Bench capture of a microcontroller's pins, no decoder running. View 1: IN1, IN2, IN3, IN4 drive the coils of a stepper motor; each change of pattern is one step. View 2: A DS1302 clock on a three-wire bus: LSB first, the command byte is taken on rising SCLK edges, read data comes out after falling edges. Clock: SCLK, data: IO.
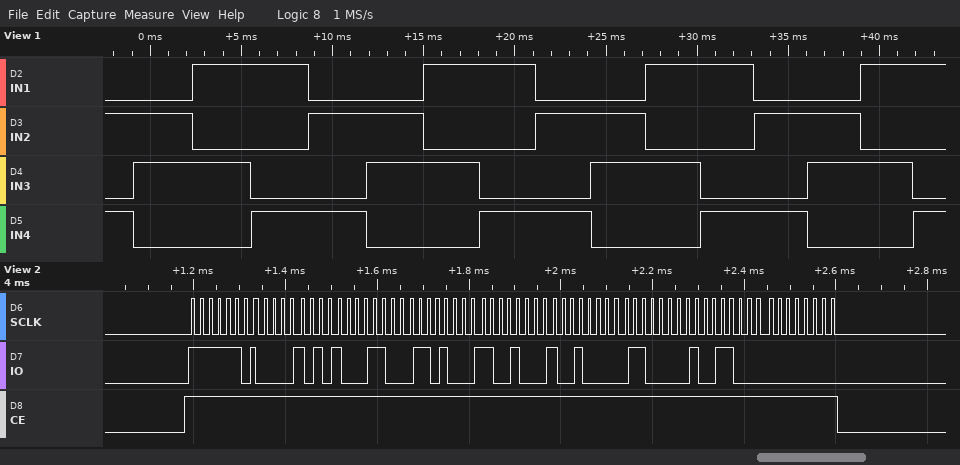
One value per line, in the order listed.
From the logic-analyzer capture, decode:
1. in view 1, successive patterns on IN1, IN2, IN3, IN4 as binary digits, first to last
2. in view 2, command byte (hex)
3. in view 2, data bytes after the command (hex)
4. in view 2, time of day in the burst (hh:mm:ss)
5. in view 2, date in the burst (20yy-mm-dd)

0101 0110 1010 1001 0101 0110 1010 1001 0101 0110 1010 1001 0101 0110 1010 1001
0xBF
50 31 16 13 09 06 19 00
16:31:50
2019-09-13
